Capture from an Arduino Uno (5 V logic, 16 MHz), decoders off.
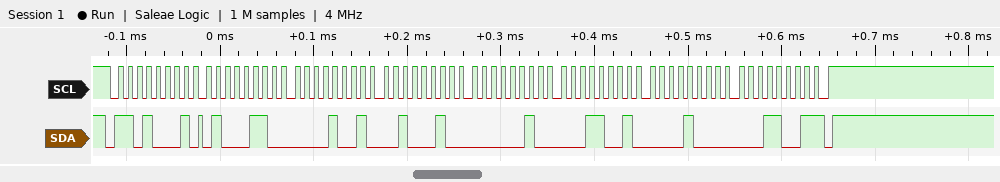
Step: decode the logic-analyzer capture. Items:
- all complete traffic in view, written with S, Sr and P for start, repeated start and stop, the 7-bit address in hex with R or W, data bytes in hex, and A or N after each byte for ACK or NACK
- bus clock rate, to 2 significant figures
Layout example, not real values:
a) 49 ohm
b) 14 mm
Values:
a) S 68R A 46 A 09 A 22 A 02 A 19 A 08 A 19 N P
b) 100 kHz
